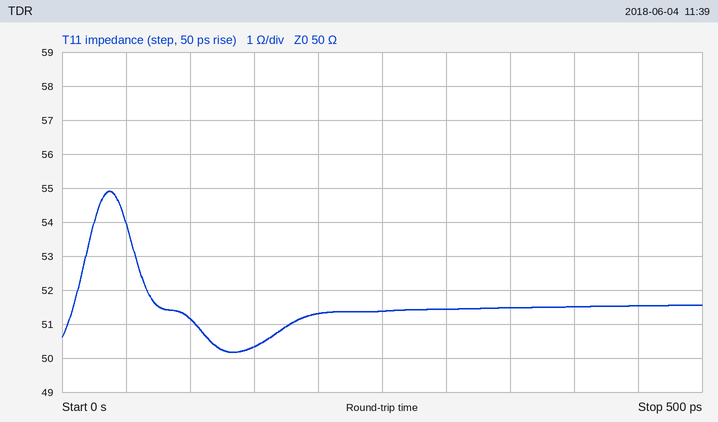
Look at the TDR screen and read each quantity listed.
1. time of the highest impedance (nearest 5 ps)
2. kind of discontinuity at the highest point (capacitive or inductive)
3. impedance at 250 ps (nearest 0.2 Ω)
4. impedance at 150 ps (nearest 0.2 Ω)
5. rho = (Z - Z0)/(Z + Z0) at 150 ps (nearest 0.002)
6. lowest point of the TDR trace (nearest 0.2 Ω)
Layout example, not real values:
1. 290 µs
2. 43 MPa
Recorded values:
1. 35 ps
2. inductive
3. 51.4 Ω
4. 50.4 Ω
5. +0.004
6. 50.2 Ω
